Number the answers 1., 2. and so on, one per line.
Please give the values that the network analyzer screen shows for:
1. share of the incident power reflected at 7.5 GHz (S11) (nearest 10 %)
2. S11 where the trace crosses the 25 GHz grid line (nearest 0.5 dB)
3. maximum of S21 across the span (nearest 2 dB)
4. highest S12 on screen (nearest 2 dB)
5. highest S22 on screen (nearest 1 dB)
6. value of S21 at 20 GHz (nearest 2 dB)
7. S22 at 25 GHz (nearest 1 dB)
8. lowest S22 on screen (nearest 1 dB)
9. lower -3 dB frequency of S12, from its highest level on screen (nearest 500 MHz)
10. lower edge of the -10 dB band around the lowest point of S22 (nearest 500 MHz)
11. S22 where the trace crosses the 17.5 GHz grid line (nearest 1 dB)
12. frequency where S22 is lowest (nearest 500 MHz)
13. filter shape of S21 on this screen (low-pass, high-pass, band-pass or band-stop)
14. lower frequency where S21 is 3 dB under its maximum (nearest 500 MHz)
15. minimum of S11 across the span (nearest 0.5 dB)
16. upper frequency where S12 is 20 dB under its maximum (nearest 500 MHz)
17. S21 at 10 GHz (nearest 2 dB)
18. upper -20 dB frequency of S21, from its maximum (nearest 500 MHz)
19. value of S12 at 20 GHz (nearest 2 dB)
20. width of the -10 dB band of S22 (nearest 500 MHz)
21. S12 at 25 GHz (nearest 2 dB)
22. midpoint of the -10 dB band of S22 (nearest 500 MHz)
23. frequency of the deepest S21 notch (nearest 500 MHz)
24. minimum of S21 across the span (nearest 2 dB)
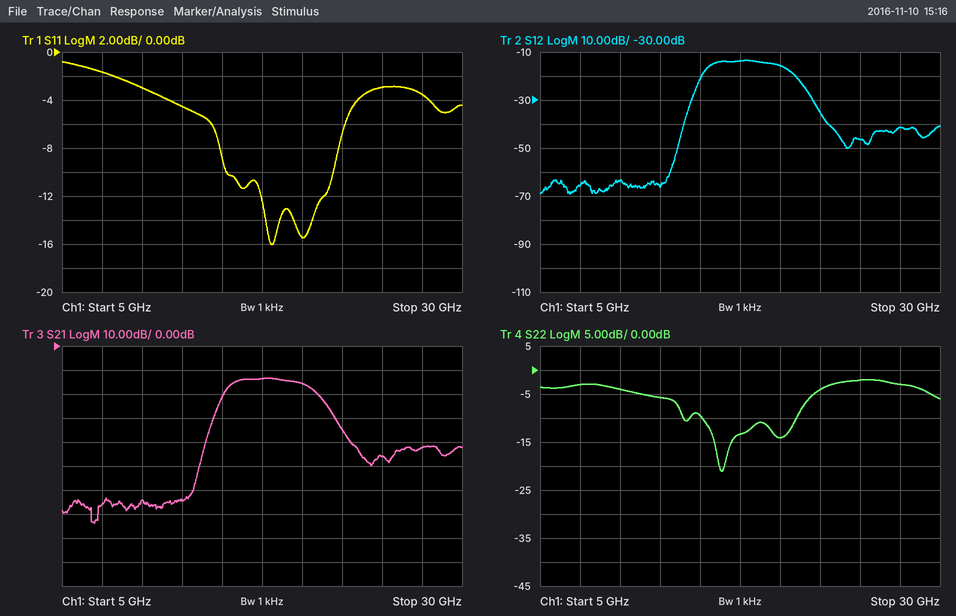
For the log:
1. 70 %
2. -3.0 dB
3. -14 dB
4. -14 dB
5. -2 dB
6. -16 dB
7. -2 dB
8. -21 dB
9. 15.5 GHz
10. 15.0 GHz
11. -13 dB
12. 16.5 GHz
13. band-pass
14. 15.5 GHz
15. -16.0 dB
16. 22.5 GHz
17. -64 dB
18. 22.5 GHz
19. -16 dB
20. 6.0 GHz
21. -46 dB
22. 18.0 GHz
23. 7.0 GHz
24. -74 dB
